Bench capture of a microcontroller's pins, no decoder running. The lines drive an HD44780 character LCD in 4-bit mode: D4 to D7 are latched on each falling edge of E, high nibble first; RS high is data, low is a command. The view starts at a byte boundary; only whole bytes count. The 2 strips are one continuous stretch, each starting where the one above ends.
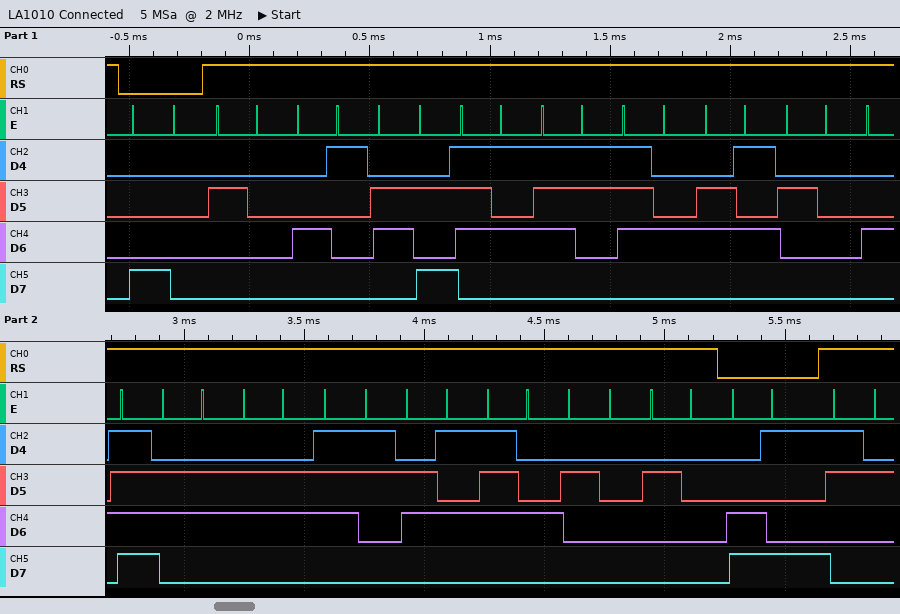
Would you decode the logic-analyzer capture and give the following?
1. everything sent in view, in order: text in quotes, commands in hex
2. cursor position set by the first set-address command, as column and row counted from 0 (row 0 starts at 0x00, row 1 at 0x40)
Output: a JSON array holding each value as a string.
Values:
["0x80 \" Ajuste Offset  \" 0xC9 \"2\"", "column 0, row 0"]
